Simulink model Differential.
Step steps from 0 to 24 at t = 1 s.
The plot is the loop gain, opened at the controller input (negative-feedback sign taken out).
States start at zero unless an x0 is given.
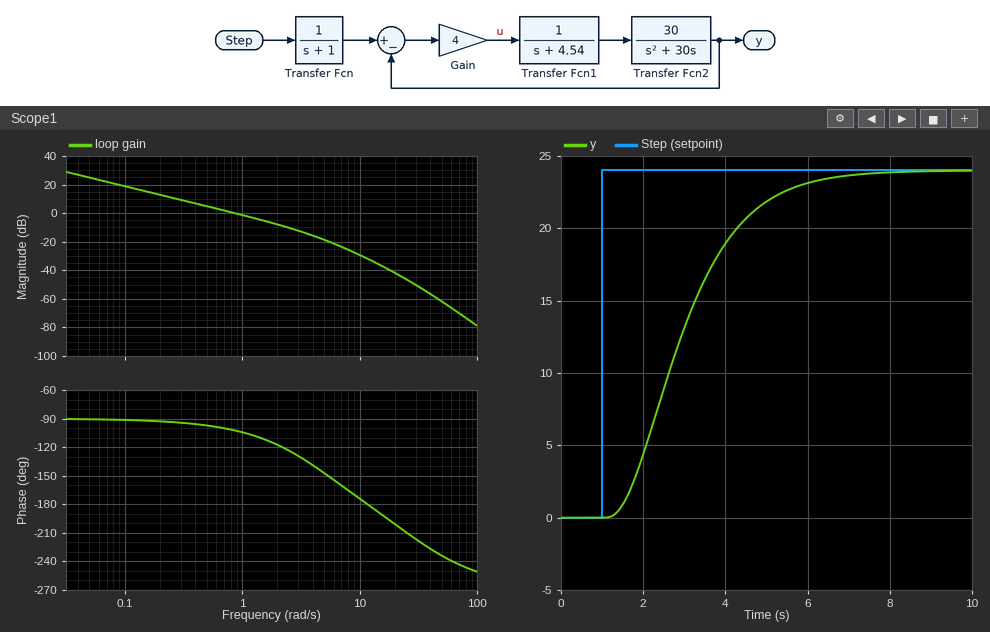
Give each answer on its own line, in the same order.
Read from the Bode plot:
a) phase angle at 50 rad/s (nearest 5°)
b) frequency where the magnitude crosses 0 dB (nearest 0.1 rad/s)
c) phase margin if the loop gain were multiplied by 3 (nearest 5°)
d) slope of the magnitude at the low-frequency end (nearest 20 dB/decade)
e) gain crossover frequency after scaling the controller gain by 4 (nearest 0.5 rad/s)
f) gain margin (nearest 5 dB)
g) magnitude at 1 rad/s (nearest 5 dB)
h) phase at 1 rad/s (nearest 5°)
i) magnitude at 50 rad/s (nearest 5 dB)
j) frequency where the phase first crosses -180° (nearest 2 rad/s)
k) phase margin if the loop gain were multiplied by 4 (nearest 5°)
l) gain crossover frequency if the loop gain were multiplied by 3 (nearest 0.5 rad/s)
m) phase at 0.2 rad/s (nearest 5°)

-235°
0.9 rad/s
60°
-20 dB/decade
3.0 rad/s
30 dB
0 dB
-105°
-60 dB
12 rad/s
50°
2.5 rad/s
-95°
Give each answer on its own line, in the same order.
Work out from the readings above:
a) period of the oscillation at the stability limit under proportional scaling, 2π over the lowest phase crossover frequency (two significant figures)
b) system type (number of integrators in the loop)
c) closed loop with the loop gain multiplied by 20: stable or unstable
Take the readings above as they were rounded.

0.52 s
1
stable
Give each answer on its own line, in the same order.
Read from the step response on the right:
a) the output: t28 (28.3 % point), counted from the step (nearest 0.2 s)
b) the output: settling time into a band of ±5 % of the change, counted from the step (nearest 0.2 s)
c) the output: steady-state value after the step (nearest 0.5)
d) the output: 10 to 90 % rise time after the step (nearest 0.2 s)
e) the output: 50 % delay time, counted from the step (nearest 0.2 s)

1.2 s
4.6 s
24.0
3.2 s
1.8 s
